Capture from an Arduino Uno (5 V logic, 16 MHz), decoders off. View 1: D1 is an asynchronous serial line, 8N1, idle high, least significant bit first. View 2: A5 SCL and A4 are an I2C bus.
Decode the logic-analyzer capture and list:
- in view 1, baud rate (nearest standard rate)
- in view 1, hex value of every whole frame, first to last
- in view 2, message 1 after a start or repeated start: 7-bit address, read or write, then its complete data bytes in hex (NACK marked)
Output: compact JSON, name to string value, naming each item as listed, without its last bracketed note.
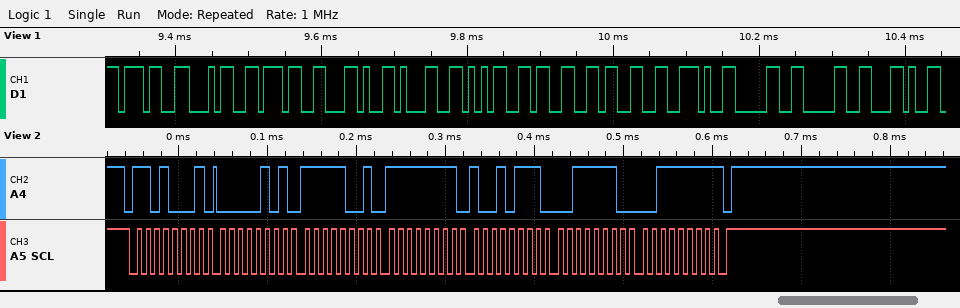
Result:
{"in view 1, baud rate": "115200 baud", "in view 1, hex value of every whole frame, first to last": "37 34 37 2C 31 35 33 33 2E 30 30 2C", "in view 2, message 1 after a start or repeated start: 7-bit address, read or write, then its complete data bytes in hex": "0x68 read: 05 F9 FF 97 3E 3F NACK"}
